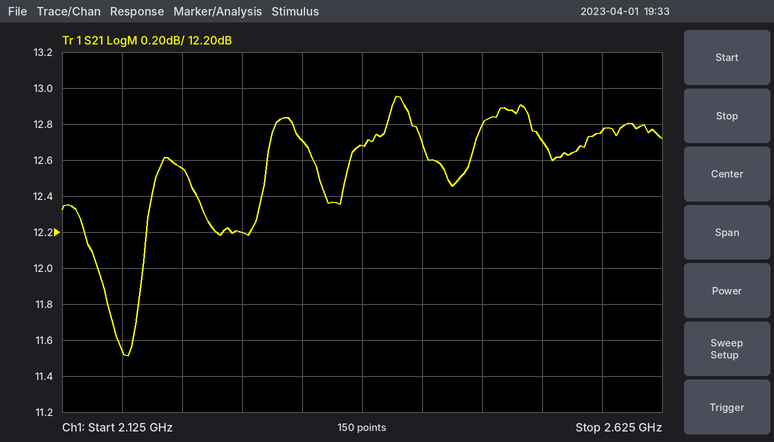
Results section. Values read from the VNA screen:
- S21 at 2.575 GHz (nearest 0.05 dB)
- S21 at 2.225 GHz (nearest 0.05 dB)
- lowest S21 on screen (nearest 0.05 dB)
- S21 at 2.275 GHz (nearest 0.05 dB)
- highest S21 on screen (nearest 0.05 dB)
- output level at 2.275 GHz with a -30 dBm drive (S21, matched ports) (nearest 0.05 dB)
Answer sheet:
12.75 dB
12.55 dB
11.50 dB
12.20 dB
12.95 dB
-17.80 dBm
